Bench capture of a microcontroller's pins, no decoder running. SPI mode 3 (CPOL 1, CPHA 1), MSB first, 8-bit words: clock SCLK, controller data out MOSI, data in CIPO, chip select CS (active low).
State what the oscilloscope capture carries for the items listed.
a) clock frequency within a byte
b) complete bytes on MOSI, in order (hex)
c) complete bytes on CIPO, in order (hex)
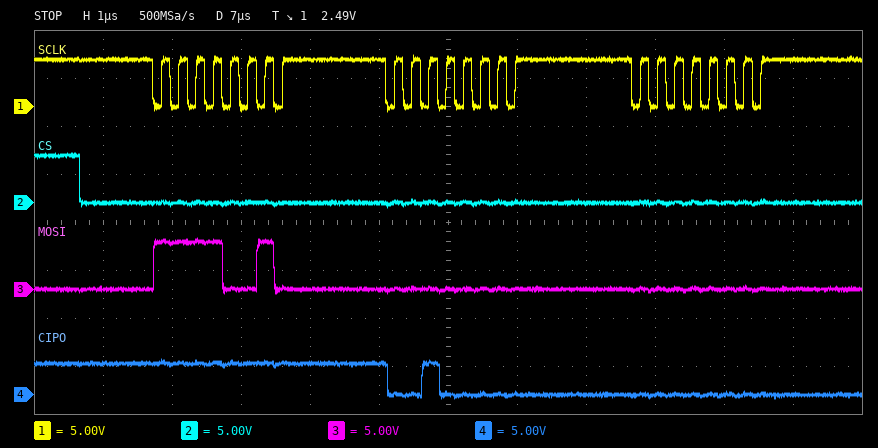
4 MHz
F2 00 00
FF 20 00
